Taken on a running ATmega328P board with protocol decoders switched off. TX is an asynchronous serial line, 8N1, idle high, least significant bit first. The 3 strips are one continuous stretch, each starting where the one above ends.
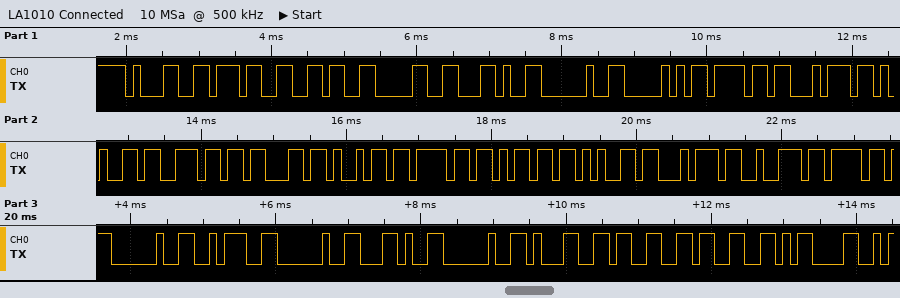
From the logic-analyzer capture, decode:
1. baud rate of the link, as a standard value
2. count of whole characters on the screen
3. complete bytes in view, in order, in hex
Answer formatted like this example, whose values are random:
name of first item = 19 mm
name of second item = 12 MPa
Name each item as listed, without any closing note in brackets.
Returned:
baud rate of the link, as a standard value = 9600 baud
count of whole characters on the screen = 28
complete bytes in view, in order, in hex = 31 37 36 30 2C 20 50 6F 74 65 6E 63 69 6F 6D 65 74 72 6F 20 3A 20 2C 20 31 33 33 0D
